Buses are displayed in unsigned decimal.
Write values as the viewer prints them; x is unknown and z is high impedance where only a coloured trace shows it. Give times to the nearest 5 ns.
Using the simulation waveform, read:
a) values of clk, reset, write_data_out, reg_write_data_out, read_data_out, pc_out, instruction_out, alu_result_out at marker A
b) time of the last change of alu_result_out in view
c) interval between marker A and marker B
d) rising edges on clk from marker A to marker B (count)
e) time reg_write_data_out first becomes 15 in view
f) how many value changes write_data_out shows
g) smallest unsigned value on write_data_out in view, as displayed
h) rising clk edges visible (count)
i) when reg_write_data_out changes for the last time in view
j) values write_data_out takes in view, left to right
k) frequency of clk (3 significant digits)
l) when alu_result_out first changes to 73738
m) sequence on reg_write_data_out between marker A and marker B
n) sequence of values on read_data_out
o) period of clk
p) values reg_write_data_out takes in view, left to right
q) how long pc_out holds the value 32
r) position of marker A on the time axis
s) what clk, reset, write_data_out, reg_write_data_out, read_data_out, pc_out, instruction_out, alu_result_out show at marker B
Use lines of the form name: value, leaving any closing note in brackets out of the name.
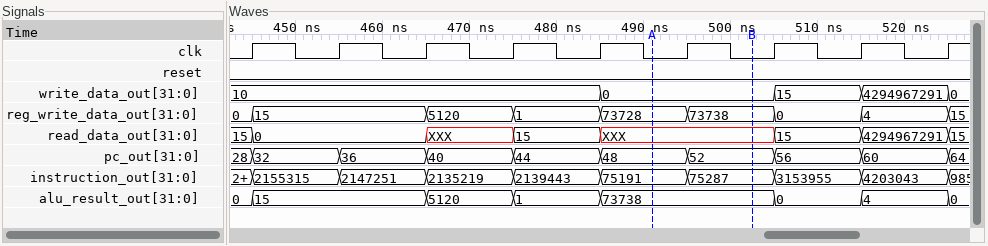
values of clk, reset, write_data_out, reg_write_data_out, read_data_out, pc_out, instruction_out, alu_result_out at marker A: clk=0, reset=0, write_data_out=0, reg_write_data_out=73728, read_data_out=XXX, pc_out=48, instruction_out=75191, alu_result_out=73738
time of the last change of alu_result_out in view: 525 ns
interval between marker A and marker B: 10 ns
rising edges on clk from marker A to marker B: 1
time reg_write_data_out first becomes 15 in view: 445 ns
how many value changes write_data_out shows: 4
smallest unsigned value on write_data_out in view, as displayed: 0
rising clk edges visible: 9
when reg_write_data_out changes for the last time in view: 525 ns
values write_data_out takes in view, left to right: 10, 0, 15, 4294967291, 0
frequency of clk: 100 MHz
when alu_result_out first changes to 73738: 485 ns
sequence on reg_write_data_out between marker A and marker B: 73728, 73738
sequence of values on read_data_out: 15, 0, XXX, 15, XXX, 15, 4294967291, 15
period of clk: 10 ns
values reg_write_data_out takes in view, left to right: 0, 15, 5120, 1, 73728, 73738, 0, 4, 15
how long pc_out holds the value 32: 10 ns
position of marker A on the time axis: 490 ns
what clk, reset, write_data_out, reg_write_data_out, read_data_out, pc_out, instruction_out, alu_result_out show at marker B: clk=0, reset=0, write_data_out=0, reg_write_data_out=73738, read_data_out=XXX, pc_out=52, instruction_out=75287, alu_result_out=73738
